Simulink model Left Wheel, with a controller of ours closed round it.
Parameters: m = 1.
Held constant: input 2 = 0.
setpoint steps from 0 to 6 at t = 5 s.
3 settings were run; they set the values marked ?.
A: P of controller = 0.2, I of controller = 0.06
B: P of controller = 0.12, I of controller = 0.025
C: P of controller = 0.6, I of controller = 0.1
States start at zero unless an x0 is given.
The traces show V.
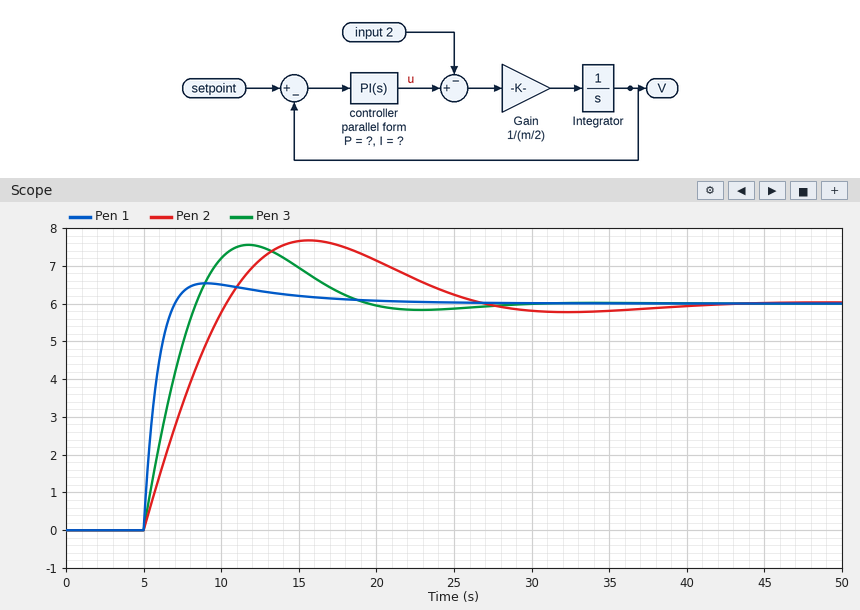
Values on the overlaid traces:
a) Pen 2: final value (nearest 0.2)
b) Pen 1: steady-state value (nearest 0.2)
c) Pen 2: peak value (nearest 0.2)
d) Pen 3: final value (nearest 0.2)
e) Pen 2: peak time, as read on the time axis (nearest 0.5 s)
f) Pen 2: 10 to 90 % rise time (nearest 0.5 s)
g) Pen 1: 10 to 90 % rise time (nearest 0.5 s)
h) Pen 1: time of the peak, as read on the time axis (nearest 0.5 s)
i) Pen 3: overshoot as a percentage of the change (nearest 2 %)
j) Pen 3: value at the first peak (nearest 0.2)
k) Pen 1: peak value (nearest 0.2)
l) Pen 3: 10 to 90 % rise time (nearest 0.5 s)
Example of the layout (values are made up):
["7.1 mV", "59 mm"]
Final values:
["6.0", "6.0", "7.6", "6.0", "15.5 s", "4.0 s", "1.5 s", "9.0 s", "26 %", "7.6", "6.6", "2.5 s"]
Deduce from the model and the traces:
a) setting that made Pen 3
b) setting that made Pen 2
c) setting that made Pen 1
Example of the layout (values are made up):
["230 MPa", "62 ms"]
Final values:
["A", "B", "C"]
